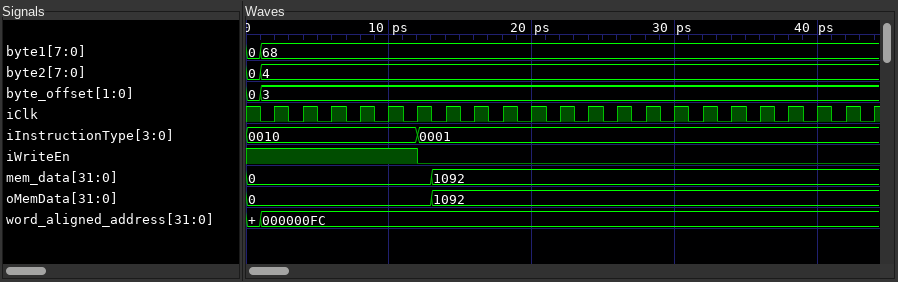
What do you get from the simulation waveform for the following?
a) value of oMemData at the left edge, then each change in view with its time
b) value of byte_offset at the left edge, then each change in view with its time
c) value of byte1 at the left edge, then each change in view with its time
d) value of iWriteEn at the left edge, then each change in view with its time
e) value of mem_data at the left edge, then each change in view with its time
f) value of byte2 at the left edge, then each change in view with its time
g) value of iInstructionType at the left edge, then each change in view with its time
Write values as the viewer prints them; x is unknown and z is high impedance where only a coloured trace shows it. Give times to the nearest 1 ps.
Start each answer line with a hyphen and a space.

- 0, 1092 at 13 ps
- 0, 3 at 1 ps
- 0, 68 at 1 ps
- 1, 0 at 12 ps
- 0, 1092 at 13 ps
- 0, 4 at 1 ps
- 0010, 0001 at 12 ps
